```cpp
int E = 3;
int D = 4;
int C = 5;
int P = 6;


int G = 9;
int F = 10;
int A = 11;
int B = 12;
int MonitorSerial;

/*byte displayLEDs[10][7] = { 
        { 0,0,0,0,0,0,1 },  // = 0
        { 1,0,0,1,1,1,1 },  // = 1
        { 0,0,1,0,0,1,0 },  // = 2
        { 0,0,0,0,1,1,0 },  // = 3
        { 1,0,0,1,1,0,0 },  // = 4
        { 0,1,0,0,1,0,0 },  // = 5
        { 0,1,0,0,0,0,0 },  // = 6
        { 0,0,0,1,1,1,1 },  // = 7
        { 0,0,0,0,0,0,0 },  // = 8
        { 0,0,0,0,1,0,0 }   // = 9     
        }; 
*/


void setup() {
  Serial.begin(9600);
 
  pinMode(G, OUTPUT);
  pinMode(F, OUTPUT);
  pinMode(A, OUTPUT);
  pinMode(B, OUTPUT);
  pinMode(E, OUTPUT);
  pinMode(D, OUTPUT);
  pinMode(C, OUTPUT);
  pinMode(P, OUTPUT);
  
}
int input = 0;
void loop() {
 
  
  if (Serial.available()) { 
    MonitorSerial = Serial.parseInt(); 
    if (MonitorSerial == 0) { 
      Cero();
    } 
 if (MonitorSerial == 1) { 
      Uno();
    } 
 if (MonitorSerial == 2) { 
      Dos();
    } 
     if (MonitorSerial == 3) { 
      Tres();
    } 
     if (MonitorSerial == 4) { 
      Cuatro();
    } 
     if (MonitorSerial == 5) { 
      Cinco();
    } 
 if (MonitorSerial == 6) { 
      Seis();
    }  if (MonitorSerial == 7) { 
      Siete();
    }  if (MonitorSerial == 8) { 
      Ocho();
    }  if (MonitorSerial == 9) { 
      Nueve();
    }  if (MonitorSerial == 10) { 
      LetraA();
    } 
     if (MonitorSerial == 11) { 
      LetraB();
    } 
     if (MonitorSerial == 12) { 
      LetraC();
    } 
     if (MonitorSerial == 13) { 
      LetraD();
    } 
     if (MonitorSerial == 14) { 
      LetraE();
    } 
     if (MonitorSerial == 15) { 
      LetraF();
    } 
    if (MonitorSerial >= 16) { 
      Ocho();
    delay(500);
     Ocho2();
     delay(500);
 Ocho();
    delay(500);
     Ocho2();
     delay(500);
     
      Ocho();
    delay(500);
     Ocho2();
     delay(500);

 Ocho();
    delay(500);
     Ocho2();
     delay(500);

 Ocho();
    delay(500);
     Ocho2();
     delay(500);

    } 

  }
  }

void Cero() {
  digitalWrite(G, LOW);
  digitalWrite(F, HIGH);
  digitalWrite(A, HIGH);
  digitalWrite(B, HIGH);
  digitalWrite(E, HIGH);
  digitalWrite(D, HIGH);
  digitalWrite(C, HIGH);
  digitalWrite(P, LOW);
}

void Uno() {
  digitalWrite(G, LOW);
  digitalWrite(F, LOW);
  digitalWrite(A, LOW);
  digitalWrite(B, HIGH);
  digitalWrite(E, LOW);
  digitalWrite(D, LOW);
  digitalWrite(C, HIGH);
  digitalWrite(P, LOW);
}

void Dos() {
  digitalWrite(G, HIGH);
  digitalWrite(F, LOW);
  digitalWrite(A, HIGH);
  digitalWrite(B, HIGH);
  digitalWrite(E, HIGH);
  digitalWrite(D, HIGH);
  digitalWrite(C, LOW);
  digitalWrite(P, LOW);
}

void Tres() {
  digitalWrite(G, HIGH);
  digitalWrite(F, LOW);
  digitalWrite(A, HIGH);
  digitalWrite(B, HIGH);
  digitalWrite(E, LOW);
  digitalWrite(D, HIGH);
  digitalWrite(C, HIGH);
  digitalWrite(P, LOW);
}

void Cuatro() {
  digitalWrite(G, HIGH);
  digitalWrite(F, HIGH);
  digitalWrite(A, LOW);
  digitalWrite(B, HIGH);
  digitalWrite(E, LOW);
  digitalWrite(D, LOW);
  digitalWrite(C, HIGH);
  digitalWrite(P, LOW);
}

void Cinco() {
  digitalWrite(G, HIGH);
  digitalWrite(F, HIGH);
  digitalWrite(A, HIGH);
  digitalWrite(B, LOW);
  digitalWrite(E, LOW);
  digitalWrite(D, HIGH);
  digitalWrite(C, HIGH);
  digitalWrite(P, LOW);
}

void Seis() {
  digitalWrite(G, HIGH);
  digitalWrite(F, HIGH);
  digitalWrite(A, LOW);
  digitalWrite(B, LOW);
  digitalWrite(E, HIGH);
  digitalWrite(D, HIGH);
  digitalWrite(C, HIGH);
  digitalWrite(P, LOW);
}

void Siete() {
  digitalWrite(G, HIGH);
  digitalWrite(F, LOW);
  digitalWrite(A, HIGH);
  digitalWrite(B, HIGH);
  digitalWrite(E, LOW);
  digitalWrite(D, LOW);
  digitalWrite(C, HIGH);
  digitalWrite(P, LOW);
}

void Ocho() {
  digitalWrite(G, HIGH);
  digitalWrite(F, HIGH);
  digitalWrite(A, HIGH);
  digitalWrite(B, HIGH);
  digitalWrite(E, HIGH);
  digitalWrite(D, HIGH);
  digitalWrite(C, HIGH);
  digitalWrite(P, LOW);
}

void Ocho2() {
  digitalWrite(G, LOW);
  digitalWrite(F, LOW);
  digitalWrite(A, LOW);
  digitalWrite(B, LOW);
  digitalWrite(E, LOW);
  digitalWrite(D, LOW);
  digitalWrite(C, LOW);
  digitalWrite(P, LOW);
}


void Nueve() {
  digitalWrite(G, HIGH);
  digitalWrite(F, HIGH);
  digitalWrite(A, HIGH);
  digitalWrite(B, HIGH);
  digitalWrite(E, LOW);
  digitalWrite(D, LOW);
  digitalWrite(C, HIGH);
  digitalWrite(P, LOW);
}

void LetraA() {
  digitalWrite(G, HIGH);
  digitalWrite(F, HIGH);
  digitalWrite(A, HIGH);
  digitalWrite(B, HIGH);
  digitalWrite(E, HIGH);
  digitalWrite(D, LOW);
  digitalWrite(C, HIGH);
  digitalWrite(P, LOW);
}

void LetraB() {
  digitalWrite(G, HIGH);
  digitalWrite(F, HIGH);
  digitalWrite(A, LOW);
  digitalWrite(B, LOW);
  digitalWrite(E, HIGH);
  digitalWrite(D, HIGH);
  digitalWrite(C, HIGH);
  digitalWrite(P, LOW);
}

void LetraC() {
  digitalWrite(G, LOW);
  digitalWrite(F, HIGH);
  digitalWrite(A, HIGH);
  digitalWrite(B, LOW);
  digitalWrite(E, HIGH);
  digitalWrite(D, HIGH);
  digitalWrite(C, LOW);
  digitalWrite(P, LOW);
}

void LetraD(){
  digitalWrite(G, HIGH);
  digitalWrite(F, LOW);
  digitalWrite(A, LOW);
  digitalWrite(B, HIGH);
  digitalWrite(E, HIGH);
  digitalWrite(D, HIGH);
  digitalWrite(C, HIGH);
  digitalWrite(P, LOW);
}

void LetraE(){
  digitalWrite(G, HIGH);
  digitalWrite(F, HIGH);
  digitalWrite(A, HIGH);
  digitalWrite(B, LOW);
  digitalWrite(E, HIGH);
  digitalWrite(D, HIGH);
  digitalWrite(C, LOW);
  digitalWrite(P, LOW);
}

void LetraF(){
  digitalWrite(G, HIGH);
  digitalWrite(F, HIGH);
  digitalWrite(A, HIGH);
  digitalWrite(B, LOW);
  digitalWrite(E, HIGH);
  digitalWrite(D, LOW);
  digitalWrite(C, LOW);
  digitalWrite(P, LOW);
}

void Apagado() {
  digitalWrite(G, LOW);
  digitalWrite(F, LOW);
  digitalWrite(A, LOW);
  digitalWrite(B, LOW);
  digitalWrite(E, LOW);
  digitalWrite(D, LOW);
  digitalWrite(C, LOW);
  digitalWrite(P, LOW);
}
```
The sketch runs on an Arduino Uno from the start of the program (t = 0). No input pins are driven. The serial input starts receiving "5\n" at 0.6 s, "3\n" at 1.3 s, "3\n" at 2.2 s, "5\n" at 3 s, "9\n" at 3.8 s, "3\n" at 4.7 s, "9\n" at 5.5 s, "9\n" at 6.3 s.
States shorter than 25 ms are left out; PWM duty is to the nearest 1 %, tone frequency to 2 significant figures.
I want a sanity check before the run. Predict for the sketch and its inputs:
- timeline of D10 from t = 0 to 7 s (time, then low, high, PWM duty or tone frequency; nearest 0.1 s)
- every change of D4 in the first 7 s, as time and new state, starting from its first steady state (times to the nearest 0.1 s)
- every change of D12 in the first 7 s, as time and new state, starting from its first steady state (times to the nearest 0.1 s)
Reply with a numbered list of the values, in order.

1. 0 s low; 0.6 s high; 1.3 s low; 3 s high; 4.7 s low; 5.5 s high
2. 0 s low; 0.6 s high; 3.8 s low; 4.7 s high; 5.5 s low
3. 0 s low; 1.3 s high; 3 s low; 3.8 s high
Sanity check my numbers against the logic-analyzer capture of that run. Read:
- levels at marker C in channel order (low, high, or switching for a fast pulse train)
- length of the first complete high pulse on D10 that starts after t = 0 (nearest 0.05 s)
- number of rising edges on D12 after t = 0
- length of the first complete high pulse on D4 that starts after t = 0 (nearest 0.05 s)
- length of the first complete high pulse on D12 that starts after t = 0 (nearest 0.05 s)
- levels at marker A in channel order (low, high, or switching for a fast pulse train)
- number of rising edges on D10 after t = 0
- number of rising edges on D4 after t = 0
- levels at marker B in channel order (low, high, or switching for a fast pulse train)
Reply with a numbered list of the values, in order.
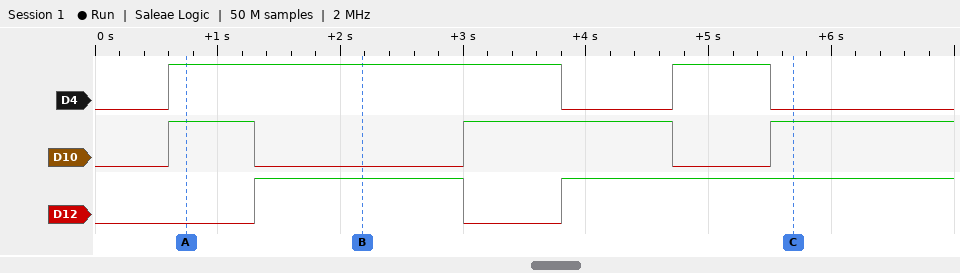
1. D4 low, D10 high, D12 high
2. 0.70 s
3. 2
4. 3.20 s
5. 1.70 s
6. D4 high, D10 high, D12 low
7. 3
8. 2
9. D4 high, D10 low, D12 high
